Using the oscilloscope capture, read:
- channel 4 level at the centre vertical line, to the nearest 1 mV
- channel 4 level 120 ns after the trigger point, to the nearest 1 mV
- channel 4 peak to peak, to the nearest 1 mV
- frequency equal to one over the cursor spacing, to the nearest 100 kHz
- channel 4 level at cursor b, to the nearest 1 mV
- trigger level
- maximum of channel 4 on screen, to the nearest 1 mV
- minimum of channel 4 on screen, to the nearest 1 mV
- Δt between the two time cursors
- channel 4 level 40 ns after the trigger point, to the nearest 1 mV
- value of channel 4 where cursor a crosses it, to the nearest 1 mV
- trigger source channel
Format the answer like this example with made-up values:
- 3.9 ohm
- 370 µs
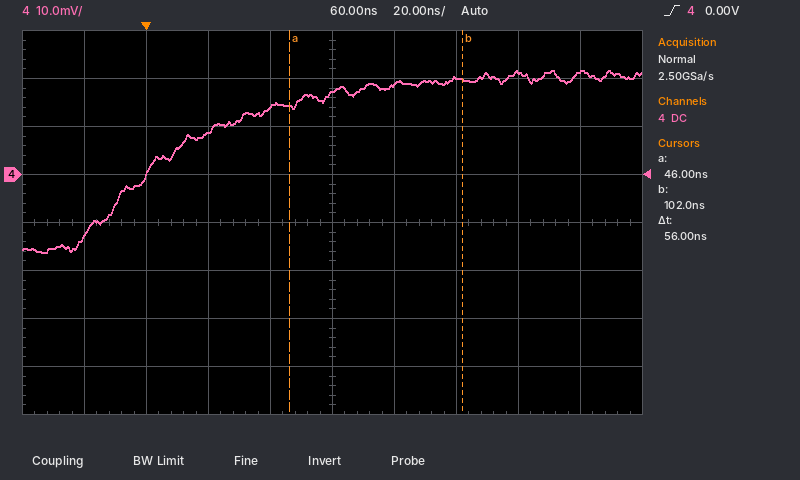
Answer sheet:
- 17 mV
- 21 mV
- 38 mV
- 17.9 MHz
- 20 mV
- 0.00 V
- 22 mV
- -16 mV
- 56 ns
- 14 mV
- 14 mV
- channel 4
